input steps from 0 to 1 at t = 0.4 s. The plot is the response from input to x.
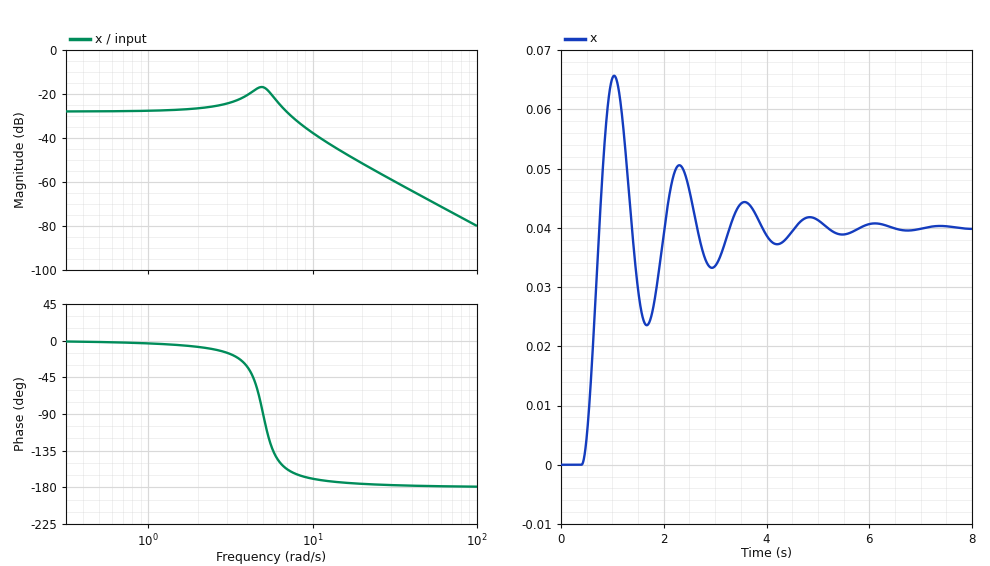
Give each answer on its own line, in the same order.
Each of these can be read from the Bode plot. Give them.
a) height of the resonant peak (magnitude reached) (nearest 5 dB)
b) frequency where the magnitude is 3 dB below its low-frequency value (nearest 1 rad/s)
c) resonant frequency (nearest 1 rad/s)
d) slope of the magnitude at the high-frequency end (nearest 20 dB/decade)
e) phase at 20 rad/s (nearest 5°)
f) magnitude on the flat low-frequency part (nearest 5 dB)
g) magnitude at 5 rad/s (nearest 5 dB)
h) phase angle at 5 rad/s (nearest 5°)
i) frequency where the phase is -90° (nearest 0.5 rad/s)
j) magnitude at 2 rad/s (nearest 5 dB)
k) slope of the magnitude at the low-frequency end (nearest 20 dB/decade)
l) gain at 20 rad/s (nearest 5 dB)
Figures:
-15 dB
8 rad/s
5 rad/s
-40 dB/decade
-175°
-30 dB
-15 dB
-90°
5.0 rad/s
-25 dB
0 dB/decade
-50 dB
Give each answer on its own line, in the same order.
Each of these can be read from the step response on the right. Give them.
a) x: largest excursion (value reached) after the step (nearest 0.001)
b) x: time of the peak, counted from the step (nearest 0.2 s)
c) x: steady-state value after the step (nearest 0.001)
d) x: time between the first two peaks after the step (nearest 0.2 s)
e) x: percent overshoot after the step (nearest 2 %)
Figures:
0.066
0.6 s
0.040
1.2 s
64 %
